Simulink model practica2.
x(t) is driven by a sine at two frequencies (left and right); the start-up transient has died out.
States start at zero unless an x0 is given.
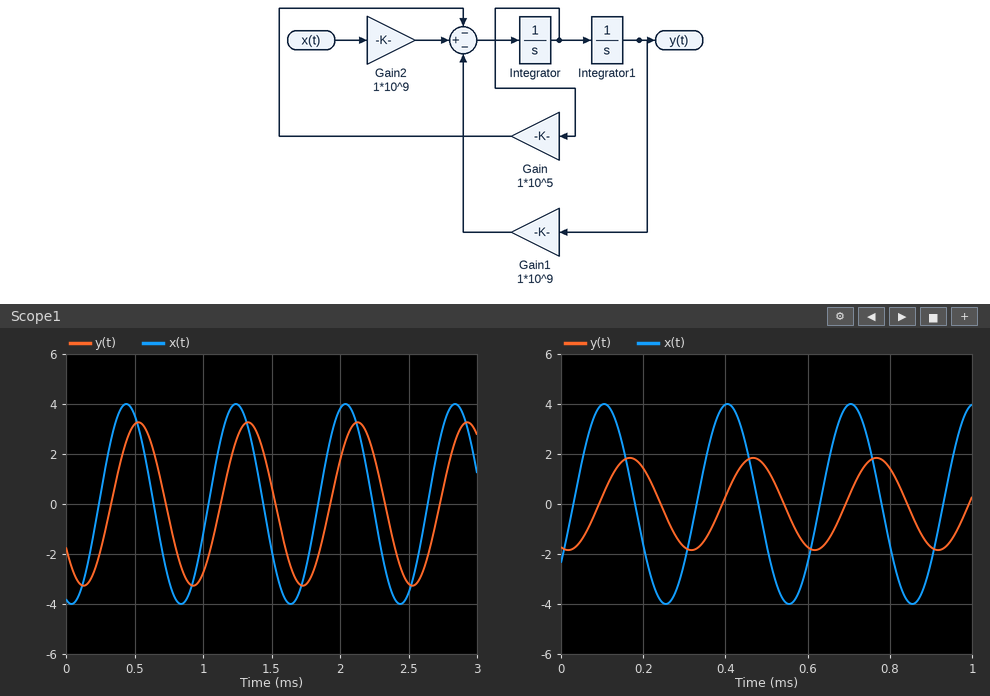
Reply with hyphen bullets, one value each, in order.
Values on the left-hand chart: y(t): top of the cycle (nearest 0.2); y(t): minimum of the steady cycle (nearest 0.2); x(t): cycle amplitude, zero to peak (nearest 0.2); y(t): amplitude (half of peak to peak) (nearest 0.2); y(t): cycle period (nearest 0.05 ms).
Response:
- 3.2
- -3.2
- 4.0
- 3.2
- 0.80 ms
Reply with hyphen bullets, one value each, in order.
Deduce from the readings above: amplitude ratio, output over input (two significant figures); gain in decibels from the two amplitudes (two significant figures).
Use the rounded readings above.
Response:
- 0.80
- -1.9 dB
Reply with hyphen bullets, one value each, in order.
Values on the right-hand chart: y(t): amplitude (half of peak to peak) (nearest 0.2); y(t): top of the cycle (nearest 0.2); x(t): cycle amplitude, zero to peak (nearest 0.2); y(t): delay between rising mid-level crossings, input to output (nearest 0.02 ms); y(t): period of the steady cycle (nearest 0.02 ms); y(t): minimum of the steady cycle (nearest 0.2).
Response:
- 1.8
- 1.8
- 4.0
- 0.06 ms
- 0.30 ms
- -1.8
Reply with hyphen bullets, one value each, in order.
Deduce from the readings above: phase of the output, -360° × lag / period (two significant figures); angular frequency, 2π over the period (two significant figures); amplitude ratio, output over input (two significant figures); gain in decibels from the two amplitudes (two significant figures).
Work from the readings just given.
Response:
- -72°
- 21 rad/ms
- 0.45
- -6.9 dB
